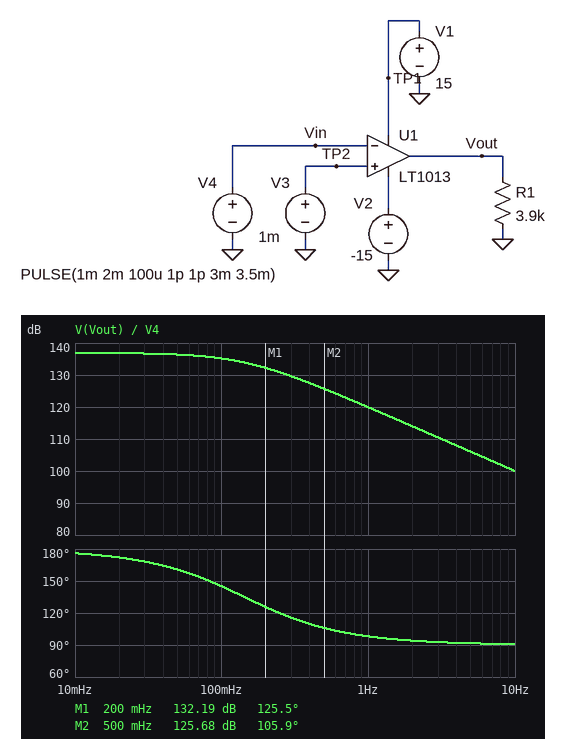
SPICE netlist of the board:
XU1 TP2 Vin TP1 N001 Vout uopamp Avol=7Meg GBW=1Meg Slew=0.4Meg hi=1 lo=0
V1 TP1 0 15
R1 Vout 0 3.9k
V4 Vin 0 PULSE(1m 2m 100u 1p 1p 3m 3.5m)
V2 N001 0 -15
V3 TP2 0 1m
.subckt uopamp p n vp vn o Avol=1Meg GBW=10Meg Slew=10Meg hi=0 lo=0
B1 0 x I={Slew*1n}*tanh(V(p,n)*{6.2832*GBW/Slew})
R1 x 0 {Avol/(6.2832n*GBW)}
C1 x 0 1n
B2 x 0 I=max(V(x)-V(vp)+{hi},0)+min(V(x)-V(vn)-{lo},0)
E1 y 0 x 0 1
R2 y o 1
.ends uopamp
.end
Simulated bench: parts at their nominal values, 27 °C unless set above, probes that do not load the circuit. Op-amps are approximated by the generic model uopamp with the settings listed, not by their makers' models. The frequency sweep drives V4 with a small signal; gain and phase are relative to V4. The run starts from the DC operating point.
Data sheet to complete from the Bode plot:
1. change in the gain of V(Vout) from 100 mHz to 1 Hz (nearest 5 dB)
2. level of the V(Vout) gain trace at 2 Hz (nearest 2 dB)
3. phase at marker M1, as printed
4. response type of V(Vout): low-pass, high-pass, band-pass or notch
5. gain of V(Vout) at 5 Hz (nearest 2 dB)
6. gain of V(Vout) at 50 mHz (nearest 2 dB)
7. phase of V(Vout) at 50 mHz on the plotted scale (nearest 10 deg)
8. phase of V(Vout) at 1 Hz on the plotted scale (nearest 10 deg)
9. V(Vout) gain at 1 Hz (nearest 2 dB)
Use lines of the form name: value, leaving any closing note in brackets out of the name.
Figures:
change in the gain of V(Vout) from 100 mHz to 1 Hz: -15 dB
level of the V(Vout) gain trace at 2 Hz: 114 dB
phase at marker M1, as printed: 125.5 deg
response type of V(Vout): low-pass, high-pass, band-pass or notch: low-pass
gain of V(Vout) at 5 Hz: 106 dB
gain of V(Vout) at 50 mHz: 136 dB
phase of V(Vout) at 50 mHz on the plotted scale: 160 deg
phase of V(Vout) at 1 Hz on the plotted scale: 100 deg
V(Vout) gain at 1 Hz: 120 dB
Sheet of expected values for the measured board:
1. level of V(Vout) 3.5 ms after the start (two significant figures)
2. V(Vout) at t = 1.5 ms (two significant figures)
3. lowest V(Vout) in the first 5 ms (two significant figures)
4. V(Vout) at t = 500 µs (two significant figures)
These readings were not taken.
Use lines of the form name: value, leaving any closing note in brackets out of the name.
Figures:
level of V(Vout) 3.5 ms after the start: -15 V
V(Vout) at t = 1.5 ms: -8.8 V
lowest V(Vout) in the first 5 ms: -15 V
V(Vout) at t = 500 µs: -2.5 V
